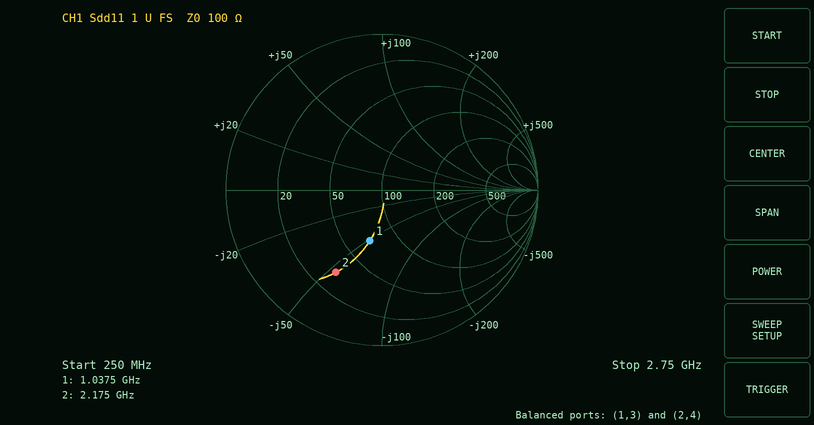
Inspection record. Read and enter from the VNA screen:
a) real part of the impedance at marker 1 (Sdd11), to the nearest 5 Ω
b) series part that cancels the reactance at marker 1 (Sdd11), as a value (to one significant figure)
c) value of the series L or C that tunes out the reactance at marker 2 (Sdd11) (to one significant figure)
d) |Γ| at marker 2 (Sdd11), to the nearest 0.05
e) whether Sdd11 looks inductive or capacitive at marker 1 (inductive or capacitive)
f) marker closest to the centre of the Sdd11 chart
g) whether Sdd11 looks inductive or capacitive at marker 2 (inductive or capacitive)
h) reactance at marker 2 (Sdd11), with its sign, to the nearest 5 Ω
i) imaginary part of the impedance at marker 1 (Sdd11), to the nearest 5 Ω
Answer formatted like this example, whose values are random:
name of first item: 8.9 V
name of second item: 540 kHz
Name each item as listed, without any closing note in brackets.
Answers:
real part of the impedance at marker 1 (Sdd11), to the nearest 5 Ω: 70 Ω
series part that cancels the reactance at marker 1 (Sdd11), as a value: 8 nH
value of the series L or C that tunes out the reactance at marker 2 (Sdd11): 4 nH
|Γ| at marker 2 (Sdd11), to the nearest 0.05: 0.60
whether Sdd11 looks inductive or capacitive at marker 1: capacitive
marker closest to the centre of the Sdd11 chart: marker 1
whether Sdd11 looks inductive or capacitive at marker 2: capacitive
reactance at marker 2 (Sdd11), with its sign, to the nearest 5 Ω: -55 Ω
imaginary part of the impedance at marker 1 (Sdd11), to the nearest 5 Ω: -50 Ω
